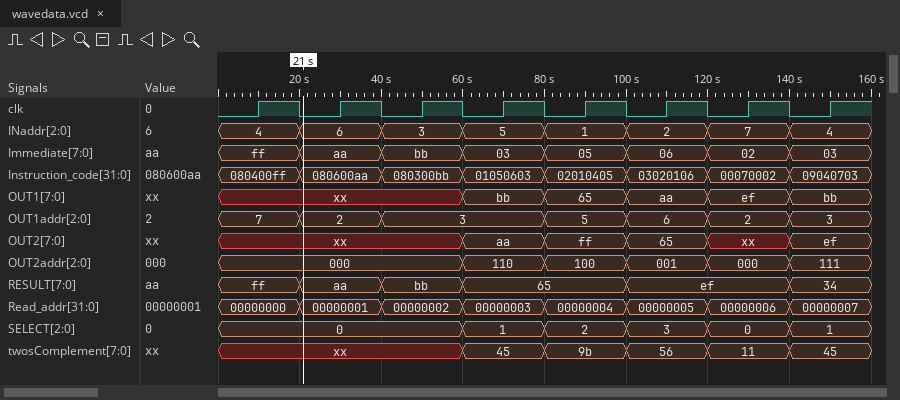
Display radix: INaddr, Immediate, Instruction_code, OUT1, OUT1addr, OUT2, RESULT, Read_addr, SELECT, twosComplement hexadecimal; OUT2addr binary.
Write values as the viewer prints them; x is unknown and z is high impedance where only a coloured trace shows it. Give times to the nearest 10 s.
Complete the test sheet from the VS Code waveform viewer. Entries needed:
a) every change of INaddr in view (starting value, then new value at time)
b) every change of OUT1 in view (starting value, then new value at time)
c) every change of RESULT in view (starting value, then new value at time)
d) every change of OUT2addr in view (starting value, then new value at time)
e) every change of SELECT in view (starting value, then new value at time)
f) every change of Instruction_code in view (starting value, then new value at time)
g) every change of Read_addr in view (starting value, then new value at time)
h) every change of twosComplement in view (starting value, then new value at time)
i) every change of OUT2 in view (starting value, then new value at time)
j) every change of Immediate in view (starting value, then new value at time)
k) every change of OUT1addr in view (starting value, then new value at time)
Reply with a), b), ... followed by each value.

a) 4, 6 at 20 s, 3 at 40 s, 5 at 60 s, 1 at 80 s, 2 at 100 s, 7 at 120 s, 4 at 140 s
b) xx, bb at 60 s, 65 at 80 s, aa at 100 s, ef at 120 s, bb at 140 s
c) ff, aa at 20 s, bb at 40 s, 65 at 60 s, ef at 100 s, 34 at 140 s
d) 000, 110 at 60 s, 100 at 80 s, 001 at 100 s, 000 at 120 s, 111 at 140 s
e) 0, 1 at 60 s, 2 at 80 s, 3 at 100 s, 0 at 120 s, 1 at 140 s
f) 080400ff, 080600aa at 20 s, 080300bb at 40 s, 01050603 at 60 s, 02010405 at 80 s, 03020106 at 100 s, 00070002 at 120 s, 09040703 at 140 s
g) 00000000, 00000001 at 20 s, 00000002 at 40 s, 00000003 at 60 s, 00000004 at 80 s, 00000005 at 100 s, 00000006 at 120 s, 00000007 at 140 s
h) xx, 45 at 60 s, 9b at 80 s, 56 at 100 s, 11 at 120 s, 45 at 140 s
i) xx, aa at 60 s, ff at 80 s, 65 at 100 s, xx at 120 s, ef at 140 s
j) ff, aa at 20 s, bb at 40 s, 03 at 60 s, 05 at 80 s, 06 at 100 s, 02 at 120 s, 03 at 140 s
k) 7, 2 at 20 s, 3 at 40 s, 5 at 80 s, 6 at 100 s, 2 at 120 s, 3 at 140 s
